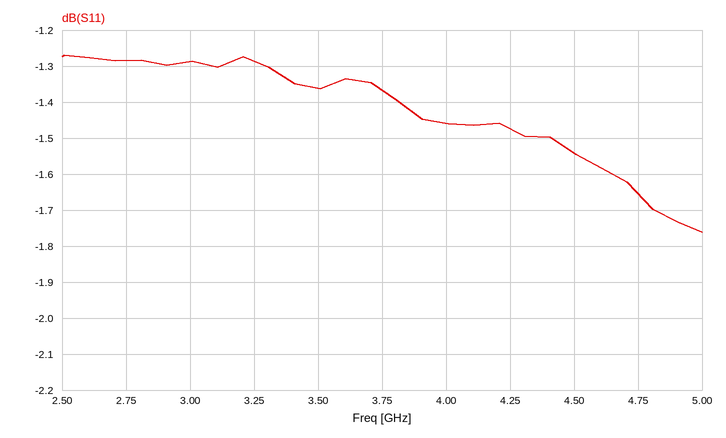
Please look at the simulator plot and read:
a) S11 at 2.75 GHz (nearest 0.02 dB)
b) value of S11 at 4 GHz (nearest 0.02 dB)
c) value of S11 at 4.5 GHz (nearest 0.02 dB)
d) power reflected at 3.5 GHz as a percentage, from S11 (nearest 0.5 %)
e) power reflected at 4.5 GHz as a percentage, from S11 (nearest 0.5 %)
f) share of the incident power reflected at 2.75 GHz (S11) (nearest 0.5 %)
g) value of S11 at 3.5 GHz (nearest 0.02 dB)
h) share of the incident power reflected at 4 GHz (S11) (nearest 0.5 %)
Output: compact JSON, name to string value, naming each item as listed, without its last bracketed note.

{"S11 at 2.75 GHz": "-1.28 dB", "value of S11 at 4 GHz": "-1.46 dB", "value of S11 at 4.5 GHz": "-1.54 dB", "power reflected at 3.5 GHz as a percentage, from S11": "73.0 %", "power reflected at 4.5 GHz as a percentage, from S11": "70.0 %", "share of the incident power reflected at 2.75 GHz (S11)": "74.5 %", "value of S11 at 3.5 GHz": "-1.36 dB", "share of the incident power reflected at 4 GHz (S11)": "71.5 %"}
